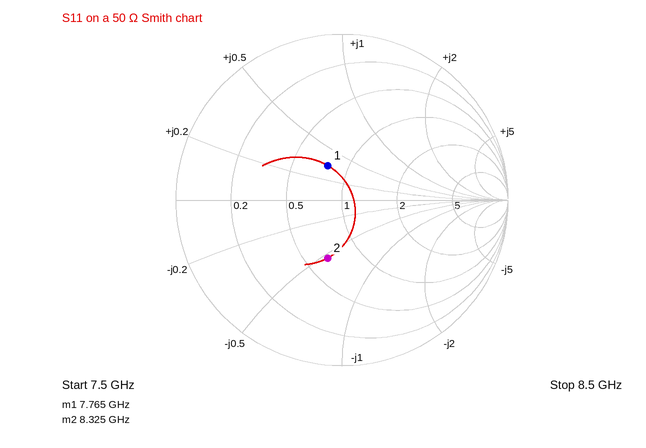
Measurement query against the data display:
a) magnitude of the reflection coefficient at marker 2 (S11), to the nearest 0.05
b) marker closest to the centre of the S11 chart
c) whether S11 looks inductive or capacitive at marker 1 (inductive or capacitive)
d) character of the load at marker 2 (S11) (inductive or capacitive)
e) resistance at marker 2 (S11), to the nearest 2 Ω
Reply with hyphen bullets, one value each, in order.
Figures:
- 0.35
- marker 1
- inductive
- capacitive
- 34 Ω
